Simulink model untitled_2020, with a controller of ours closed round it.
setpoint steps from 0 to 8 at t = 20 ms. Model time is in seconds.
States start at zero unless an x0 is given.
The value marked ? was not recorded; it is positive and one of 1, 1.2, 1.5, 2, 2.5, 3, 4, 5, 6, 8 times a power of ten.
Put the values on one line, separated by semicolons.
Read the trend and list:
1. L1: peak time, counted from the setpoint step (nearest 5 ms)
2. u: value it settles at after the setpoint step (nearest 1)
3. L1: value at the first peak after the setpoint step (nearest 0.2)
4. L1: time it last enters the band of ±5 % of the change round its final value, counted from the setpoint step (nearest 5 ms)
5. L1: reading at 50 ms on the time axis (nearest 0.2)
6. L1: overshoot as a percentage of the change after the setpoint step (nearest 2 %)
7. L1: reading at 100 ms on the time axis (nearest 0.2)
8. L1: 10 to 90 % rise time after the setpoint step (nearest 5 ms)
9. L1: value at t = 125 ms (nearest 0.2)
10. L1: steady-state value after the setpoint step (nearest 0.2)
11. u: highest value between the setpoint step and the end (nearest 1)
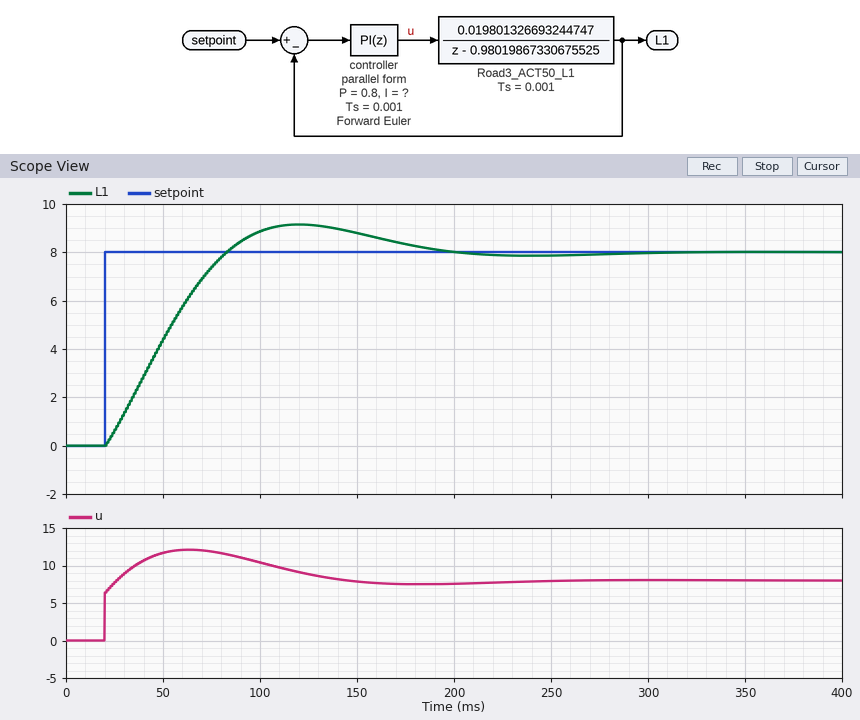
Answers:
100 ms; 8; 9.2; 150 ms; 4.4; 14 %; 8.8; 45 ms; 9.2; 8.0; 12
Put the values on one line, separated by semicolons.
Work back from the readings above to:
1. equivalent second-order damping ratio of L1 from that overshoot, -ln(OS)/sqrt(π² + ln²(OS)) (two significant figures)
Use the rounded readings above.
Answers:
0.53
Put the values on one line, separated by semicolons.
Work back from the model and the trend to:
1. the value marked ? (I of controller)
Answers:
50
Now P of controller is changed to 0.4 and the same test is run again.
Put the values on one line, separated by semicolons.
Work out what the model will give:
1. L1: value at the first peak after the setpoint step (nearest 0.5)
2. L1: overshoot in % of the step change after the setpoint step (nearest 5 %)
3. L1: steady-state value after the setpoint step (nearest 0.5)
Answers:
10.0; 25 %; 8.0
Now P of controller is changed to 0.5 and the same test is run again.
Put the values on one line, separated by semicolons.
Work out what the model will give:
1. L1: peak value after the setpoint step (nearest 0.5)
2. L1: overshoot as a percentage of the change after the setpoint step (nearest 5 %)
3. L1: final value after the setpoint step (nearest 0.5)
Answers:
9.5; 20 %; 8.0
